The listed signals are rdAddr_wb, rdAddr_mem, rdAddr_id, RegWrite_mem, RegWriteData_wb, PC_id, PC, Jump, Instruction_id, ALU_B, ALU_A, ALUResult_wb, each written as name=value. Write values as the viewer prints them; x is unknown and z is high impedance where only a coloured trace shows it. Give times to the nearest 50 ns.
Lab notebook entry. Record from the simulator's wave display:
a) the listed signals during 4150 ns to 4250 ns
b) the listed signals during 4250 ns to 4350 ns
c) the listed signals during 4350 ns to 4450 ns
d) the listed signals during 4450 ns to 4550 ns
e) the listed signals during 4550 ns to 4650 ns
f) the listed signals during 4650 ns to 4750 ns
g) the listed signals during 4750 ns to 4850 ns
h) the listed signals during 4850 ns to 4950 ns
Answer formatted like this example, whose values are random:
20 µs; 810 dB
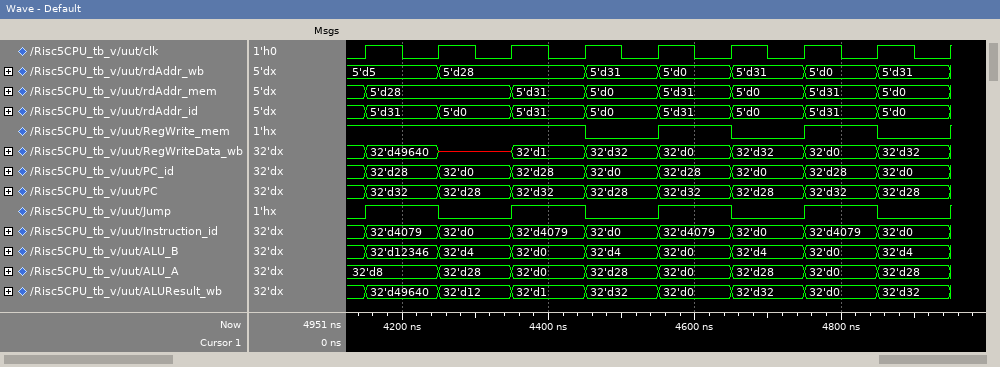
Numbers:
rdAddr_wb=5'd5, rdAddr_mem=5'd28, rdAddr_id=5'd31, RegWrite_mem=1, RegWriteData_wb=32'd49640, PC_id=32'd28, PC=32'd32, Jump=1, Instruction_id=32'd4079, ALU_B=32'd12346, ALU_A=32'd8, ALUResult_wb=32'd49640; rdAddr_wb=5'd28, rdAddr_mem=5'd28, rdAddr_id=5'd0, RegWrite_mem=1, RegWriteData_wb=x, PC_id=32'd0, PC=32'd28, Jump=0, Instruction_id=32'd0, ALU_B=32'd4, ALU_A=32'd28, ALUResult_wb=32'd12; rdAddr_wb=5'd28, rdAddr_mem=5'd31, rdAddr_id=5'd31, RegWrite_mem=1, RegWriteData_wb=32'd1, PC_id=32'd28, PC=32'd32, Jump=1, Instruction_id=32'd4079, ALU_B=32'd0, ALU_A=32'd0, ALUResult_wb=32'd1; rdAddr_wb=5'd31, rdAddr_mem=5'd0, rdAddr_id=5'd0, RegWrite_mem=0, RegWriteData_wb=32'd32, PC_id=32'd0, PC=32'd28, Jump=0, Instruction_id=32'd0, ALU_B=32'd4, ALU_A=32'd28, ALUResult_wb=32'd32; rdAddr_wb=5'd0, rdAddr_mem=5'd31, rdAddr_id=5'd31, RegWrite_mem=1, RegWriteData_wb=32'd0, PC_id=32'd28, PC=32'd32, Jump=1, Instruction_id=32'd4079, ALU_B=32'd0, ALU_A=32'd0, ALUResult_wb=32'd0; rdAddr_wb=5'd31, rdAddr_mem=5'd0, rdAddr_id=5'd0, RegWrite_mem=0, RegWriteData_wb=32'd32, PC_id=32'd0, PC=32'd28, Jump=0, Instruction_id=32'd0, ALU_B=32'd4, ALU_A=32'd28, ALUResult_wb=32'd32; rdAddr_wb=5'd0, rdAddr_mem=5'd31, rdAddr_id=5'd31, RegWrite_mem=1, RegWriteData_wb=32'd0, PC_id=32'd28, PC=32'd32, Jump=1, Instruction_id=32'd4079, ALU_B=32'd0, ALU_A=32'd0, ALUResult_wb=32'd0; rdAddr_wb=5'd31, rdAddr_mem=5'd0, rdAddr_id=5'd0, RegWrite_mem=0, RegWriteData_wb=32'd32, PC_id=32'd0, PC=32'd28, Jump=0, Instruction_id=32'd0, ALU_B=32'd4, ALU_A=32'd28, ALUResult_wb=32'd32
